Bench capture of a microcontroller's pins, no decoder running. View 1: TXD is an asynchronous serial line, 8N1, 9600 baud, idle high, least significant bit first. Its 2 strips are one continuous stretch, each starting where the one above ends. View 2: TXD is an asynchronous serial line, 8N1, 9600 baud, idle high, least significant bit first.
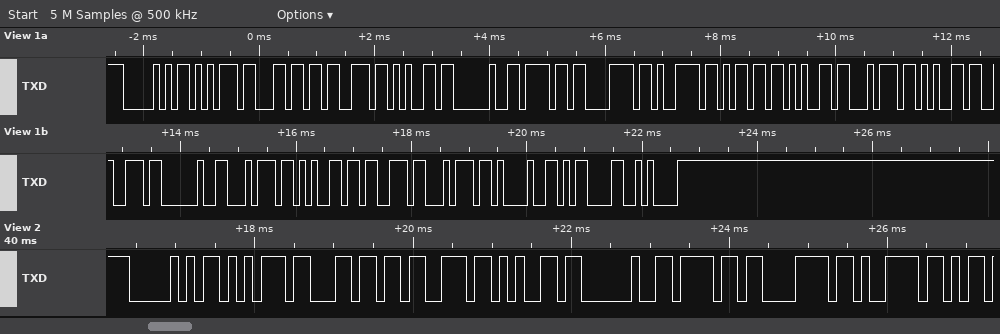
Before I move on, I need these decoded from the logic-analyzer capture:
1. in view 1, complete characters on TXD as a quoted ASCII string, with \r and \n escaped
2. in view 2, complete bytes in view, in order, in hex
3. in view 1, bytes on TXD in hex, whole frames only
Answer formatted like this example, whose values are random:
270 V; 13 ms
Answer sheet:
"Pulse oxymeter test!\r\n"; 50 75 6C 73 65 20 6F 78 79; 0x50 0x75 0x6C 0x73 0x65 0x20 0x6F 0x78 0x79 0x6D 0x65 0x74 0x65 0x72 0x20 0x74 0x65 0x73 0x74 0x21 0x0D 0x0A
